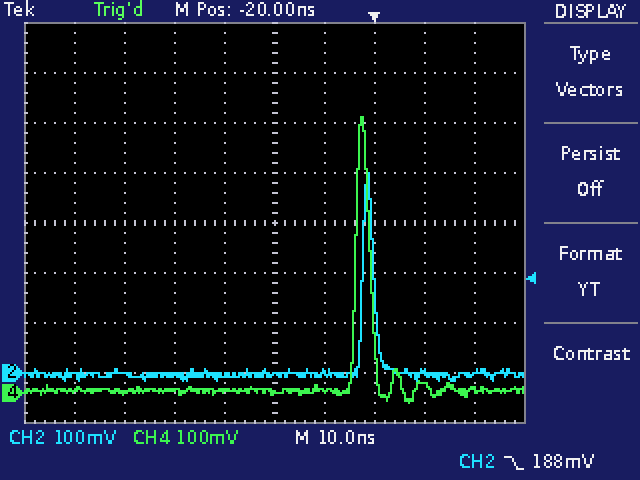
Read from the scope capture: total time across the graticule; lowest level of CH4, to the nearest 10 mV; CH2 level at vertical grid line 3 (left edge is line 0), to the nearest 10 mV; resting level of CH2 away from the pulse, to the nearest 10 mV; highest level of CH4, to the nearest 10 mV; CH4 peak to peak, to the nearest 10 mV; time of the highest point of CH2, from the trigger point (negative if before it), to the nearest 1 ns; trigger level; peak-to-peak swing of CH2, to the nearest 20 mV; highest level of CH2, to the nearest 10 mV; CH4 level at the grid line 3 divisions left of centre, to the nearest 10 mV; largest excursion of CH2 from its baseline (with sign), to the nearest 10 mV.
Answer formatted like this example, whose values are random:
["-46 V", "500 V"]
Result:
["100 ns", "-20 mV", "0 mV", "0 mV", "550 mV", "570 mV", "-1 ns", "188 mV", "420 mV", "400 mV", "0 mV", "+400 mV"]
